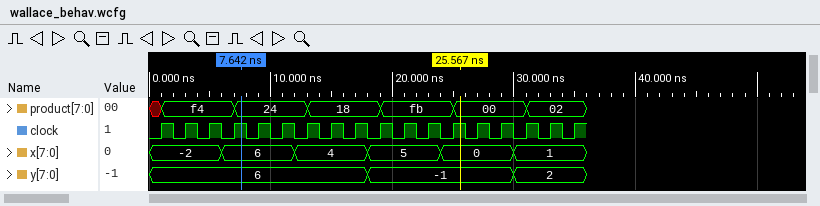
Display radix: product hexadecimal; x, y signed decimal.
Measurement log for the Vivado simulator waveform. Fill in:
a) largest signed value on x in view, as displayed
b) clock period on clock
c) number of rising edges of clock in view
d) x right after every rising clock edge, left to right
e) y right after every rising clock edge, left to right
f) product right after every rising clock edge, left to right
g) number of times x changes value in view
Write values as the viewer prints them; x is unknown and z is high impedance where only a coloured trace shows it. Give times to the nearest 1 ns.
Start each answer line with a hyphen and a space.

- 6
- 2 ns
- 18
- -2, -2, -2, 6, 6, 6, 4, 4, 4, 5, 5, 5, 0, 0, 0, 1, 1, 1
- 6, 6, 6, 6, 6, 6, 6, 6, 6, -1, -1, -1, -1, -1, -1, 2, 2, 2
- f4, f4, f4, 24, 24, 24, 18, 18, 18, fb, fb, fb, 00, 00, 00, 02, 02, 02
- 5
